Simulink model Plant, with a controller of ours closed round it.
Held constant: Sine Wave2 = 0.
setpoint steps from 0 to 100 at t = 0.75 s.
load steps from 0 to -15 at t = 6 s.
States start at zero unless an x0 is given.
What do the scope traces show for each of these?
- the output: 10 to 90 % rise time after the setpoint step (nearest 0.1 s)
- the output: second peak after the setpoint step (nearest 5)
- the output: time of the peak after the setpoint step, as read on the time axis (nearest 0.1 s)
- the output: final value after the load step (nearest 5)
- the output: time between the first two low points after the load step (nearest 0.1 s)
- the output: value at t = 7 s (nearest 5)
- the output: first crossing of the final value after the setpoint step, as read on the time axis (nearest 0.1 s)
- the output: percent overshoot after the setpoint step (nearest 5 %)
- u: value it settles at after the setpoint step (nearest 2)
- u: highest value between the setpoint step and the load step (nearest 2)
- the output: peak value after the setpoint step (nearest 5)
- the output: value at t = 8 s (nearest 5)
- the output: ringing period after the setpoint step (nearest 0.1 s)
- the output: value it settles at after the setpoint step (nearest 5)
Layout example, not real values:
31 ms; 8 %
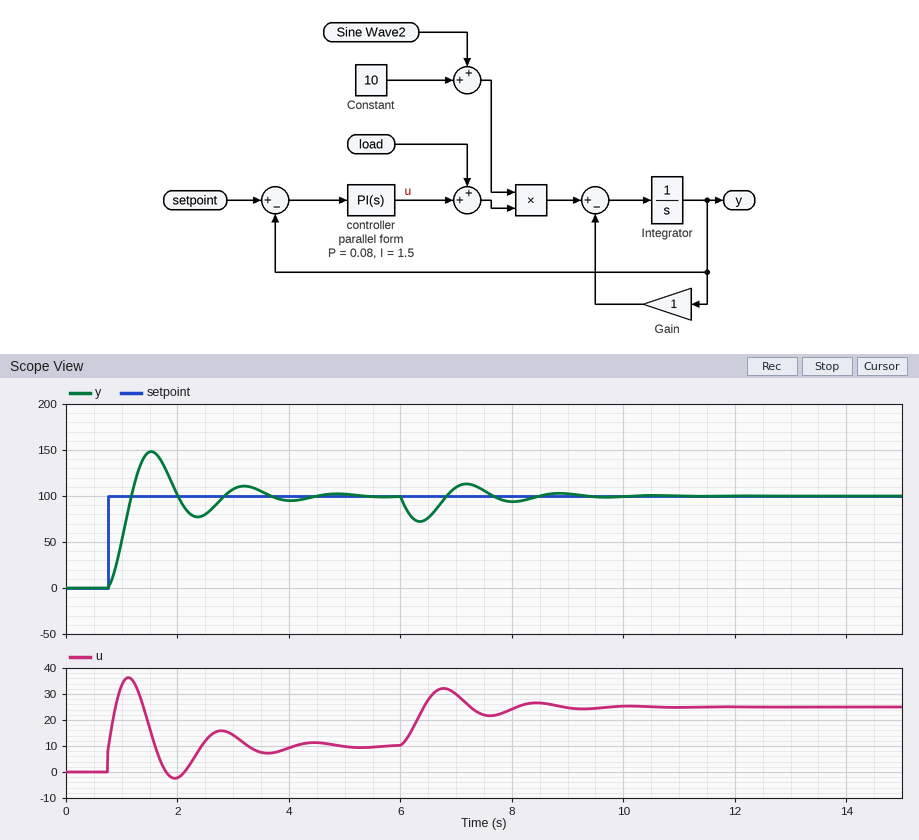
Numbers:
0.3 s; 110; 1.5 s; 100; 1.7 s; 110; 1.2 s; 50 %; 10; 36; 150; 95; 1.7 s; 100
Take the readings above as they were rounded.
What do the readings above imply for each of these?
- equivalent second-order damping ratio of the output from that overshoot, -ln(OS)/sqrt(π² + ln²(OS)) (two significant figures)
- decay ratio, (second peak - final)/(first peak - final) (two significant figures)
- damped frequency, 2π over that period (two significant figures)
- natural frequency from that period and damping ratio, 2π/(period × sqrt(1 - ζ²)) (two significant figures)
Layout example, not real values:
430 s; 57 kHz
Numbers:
0.22; 0.20; 3.7 rad/s; 3.8 rad/s
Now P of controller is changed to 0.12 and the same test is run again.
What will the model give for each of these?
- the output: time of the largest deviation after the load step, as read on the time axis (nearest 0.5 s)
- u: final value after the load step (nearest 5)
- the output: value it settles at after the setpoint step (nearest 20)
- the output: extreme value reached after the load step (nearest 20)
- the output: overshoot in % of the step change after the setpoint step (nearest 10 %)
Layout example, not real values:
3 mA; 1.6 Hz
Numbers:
6.5 s; 25; 100; 80; 40 %
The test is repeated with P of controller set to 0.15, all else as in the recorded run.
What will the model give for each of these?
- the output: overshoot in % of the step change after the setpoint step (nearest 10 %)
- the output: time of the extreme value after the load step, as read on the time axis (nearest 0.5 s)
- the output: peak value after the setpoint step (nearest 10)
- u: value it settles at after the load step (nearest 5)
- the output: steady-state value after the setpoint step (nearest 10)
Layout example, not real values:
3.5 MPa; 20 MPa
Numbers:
40 %; 6.5 s; 140; 25; 100
